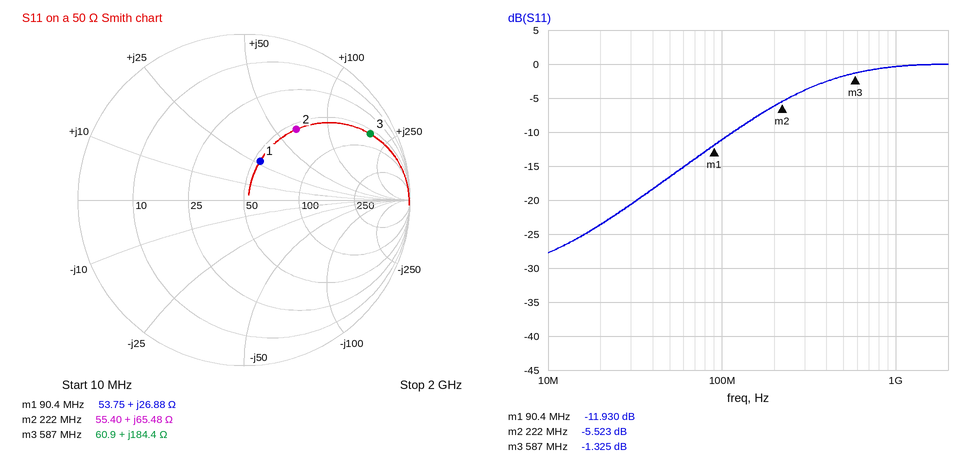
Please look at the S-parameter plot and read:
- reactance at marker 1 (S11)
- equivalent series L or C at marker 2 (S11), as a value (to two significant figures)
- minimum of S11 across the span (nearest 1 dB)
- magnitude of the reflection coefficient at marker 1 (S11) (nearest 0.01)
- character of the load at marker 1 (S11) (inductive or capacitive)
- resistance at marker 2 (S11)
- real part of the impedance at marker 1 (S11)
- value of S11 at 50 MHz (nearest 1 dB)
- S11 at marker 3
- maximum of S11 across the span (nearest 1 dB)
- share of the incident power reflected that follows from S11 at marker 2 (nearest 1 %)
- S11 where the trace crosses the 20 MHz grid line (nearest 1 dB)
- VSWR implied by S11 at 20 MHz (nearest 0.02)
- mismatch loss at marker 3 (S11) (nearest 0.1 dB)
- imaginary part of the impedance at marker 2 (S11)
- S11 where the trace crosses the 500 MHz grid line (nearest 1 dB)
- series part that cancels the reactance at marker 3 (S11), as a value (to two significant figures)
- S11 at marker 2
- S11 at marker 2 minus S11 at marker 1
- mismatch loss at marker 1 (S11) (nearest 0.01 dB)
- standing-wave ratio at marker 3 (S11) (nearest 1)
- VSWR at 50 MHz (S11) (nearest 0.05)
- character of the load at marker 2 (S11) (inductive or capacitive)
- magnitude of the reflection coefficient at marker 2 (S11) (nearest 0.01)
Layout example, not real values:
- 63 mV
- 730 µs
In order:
- +26.88 Ω
- 47 nH
- -28 dB
- 0.25
- inductive
- 55.40 Ω
- 53.75 Ω
- -17 dB
- -1.325 dB
- 0 dB
- 28 %
- -24 dB
- 1.14
- 5.8 dB
- +65.48 Ω
- -2 dB
- 1.5 pF
- -5.523 dB
- 6.407 dB
- 0.29 dB
- 13
- 1.35
- inductive
- 0.53
